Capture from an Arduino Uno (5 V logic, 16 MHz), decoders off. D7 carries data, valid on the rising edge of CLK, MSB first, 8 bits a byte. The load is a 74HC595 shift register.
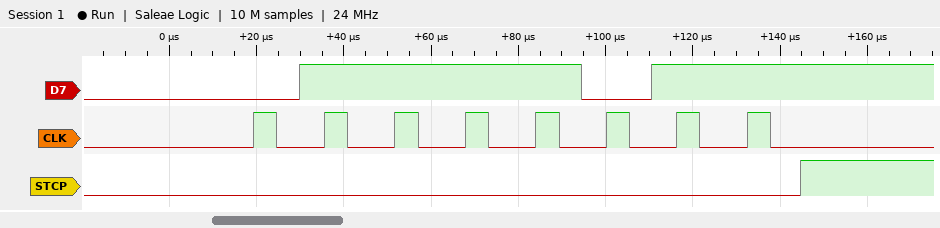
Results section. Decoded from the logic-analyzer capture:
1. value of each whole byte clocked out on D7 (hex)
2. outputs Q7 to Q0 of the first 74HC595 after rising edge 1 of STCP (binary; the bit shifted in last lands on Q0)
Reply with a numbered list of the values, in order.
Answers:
1. 7B
2. 01111011
